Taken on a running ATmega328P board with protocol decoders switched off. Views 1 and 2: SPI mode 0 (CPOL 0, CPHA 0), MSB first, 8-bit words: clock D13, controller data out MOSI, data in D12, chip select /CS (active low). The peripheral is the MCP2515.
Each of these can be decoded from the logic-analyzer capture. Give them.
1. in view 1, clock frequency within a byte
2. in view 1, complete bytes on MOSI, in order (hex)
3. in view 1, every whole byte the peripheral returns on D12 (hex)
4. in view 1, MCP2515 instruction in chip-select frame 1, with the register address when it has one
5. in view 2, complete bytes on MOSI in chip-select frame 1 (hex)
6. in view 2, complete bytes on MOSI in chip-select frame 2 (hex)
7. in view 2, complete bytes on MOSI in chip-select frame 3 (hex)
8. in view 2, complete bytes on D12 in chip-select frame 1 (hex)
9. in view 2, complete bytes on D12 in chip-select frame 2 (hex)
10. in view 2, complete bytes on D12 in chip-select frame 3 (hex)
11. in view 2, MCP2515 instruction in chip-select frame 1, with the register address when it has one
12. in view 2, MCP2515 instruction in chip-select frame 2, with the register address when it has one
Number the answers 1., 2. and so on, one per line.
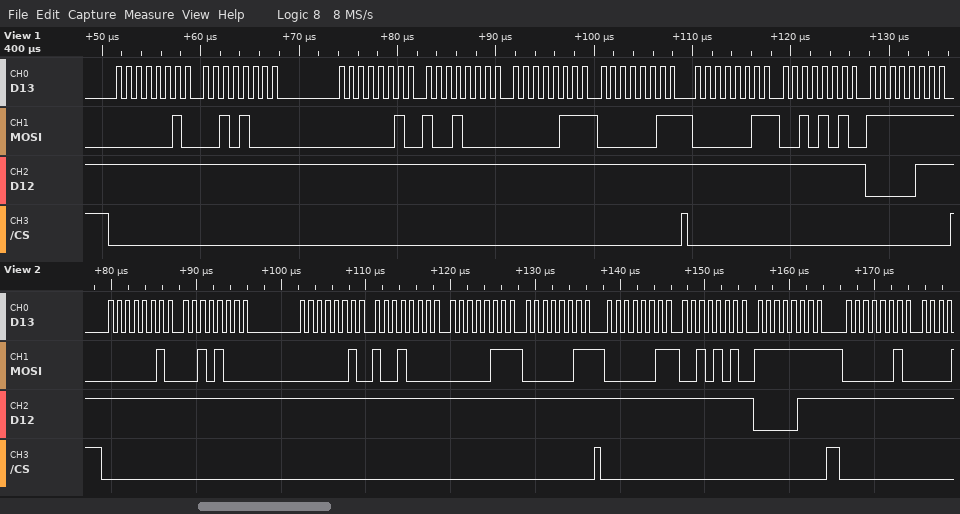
1. 1 MHz
2. 02 28 02 90 07 03 03 2A FF
3. FF FF FF FF FF FF FF FF 07
4. WRITE 0x28
5. 02 28 02 90 07 03
6. 03 2A FF
7. 02
8. FF FF FF FF FF FF
9. FF FF 07
10. FF
11. WRITE 0x28
12. READ 0x2A
